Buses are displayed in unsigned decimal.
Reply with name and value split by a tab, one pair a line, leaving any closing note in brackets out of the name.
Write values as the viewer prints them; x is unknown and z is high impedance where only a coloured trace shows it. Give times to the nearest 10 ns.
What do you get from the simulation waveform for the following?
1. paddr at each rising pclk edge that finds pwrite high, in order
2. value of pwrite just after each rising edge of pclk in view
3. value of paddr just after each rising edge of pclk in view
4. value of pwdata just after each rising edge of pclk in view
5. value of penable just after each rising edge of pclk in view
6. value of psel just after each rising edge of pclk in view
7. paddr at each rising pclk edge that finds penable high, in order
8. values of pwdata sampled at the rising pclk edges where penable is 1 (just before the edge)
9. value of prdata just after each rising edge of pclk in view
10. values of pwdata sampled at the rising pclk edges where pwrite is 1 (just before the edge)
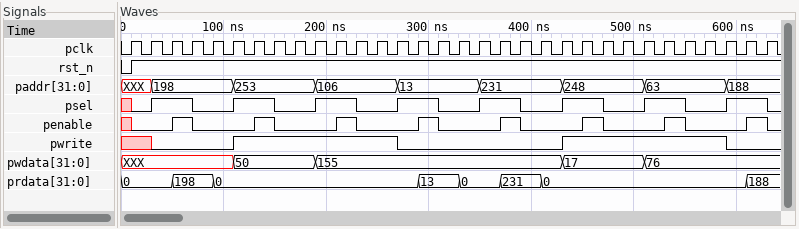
paddr at each rising pclk edge that finds pwrite high, in order	253, 253, 253, 253, 106, 106, 106, 106, 248, 248, 248, 248, 63, 63, 63, 63
value of pwrite just after each rising edge of pclk in view	x 0 0 0 0 1 1 1 1 1 1 1 1 0 0 0 0 0 0 0 0 1 1 1 1 1 1 1 1 0 0 0
value of paddr just after each rising edge of pclk in view	XXX, 198, 198, 198, 198, 253, 253, 253, 253, 106, 106, 106, 106, 13, 13, 13, 13, 231, 231, 231, 231, 248, 248, 248, 248, 63, 63, 63, 63, 188, 188, 188
value of pwdata just after each rising edge of pclk in view	XXX, XXX, XXX, XXX, XXX, 50, 50, 50, 50, 155, 155, 155, 155, 155, 155, 155, 155, 155, 155, 155, 155, 17, 17, 17, 17, 76, 76, 76, 76, 76, 76, 76
value of penable just after each rising edge of pclk in view	0 0 1 0 0 0 1 0 0 0 1 0 0 0 1 0 0 0 1 0 0 0 1 0 0 0 1 0 0 0 1 0
value of psel just after each rising edge of pclk in view	0 1 1 0 0 1 1 0 0 1 1 0 0 1 1 0 0 1 1 0 0 1 1 0 0 1 1 0 0 1 1 0
paddr at each rising pclk edge that finds penable high, in order	198, 253, 106, 13, 231, 248, 63, 188
values of pwdata sampled at the rising pclk edges where penable is 1	XXX, 50, 155, 155, 155, 17, 76, 76
value of prdata just after each rising edge of pclk in view	0, 0, 198, 198, 0, 0, 0, 0, 0, 0, 0, 0, 0, 0, 13, 13, 0, 0, 231, 231, 0, 0, 0, 0, 0, 0, 0, 0, 0, 0, 188, 188
values of pwdata sampled at the rising pclk edges where pwrite is 1	50, 50, 50, 50, 155, 155, 155, 155, 17, 17, 17, 17, 76, 76, 76, 76
